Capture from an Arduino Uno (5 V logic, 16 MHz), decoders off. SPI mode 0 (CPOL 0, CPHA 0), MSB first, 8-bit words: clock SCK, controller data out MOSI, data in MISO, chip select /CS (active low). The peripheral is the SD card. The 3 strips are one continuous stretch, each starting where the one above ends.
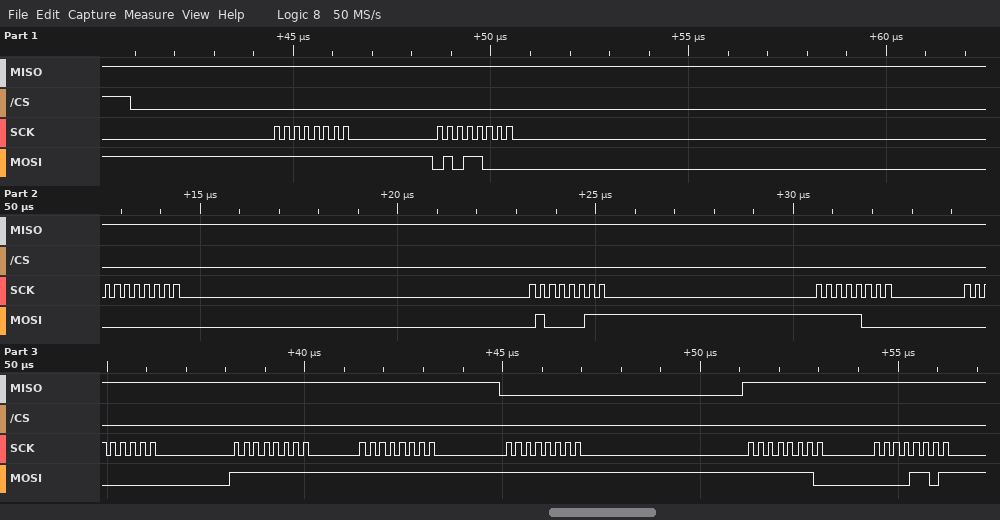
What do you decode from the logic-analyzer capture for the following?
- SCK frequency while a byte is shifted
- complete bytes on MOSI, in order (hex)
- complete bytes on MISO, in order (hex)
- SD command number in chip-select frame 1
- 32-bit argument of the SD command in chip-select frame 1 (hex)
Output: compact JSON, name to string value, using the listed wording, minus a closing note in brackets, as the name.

{"SCK frequency while a byte is shifted": "4 MHz", "complete bytes on MOSI, in order": "0xFF 0x58 0x00 0x43 0xF8 0x00 0xFF 0xFF 0xFF 0xFE 0x0D", "complete bytes on MISO, in order": "0xFF 0xFF 0xFF 0xFF 0xFF 0xFF 0xFF 0xFF 0x00 0xFF 0xFF", "SD command number in chip-select frame 1": "CMD24", "32-bit argument of the SD command in chip-select frame 1": "0x0043F800"}
